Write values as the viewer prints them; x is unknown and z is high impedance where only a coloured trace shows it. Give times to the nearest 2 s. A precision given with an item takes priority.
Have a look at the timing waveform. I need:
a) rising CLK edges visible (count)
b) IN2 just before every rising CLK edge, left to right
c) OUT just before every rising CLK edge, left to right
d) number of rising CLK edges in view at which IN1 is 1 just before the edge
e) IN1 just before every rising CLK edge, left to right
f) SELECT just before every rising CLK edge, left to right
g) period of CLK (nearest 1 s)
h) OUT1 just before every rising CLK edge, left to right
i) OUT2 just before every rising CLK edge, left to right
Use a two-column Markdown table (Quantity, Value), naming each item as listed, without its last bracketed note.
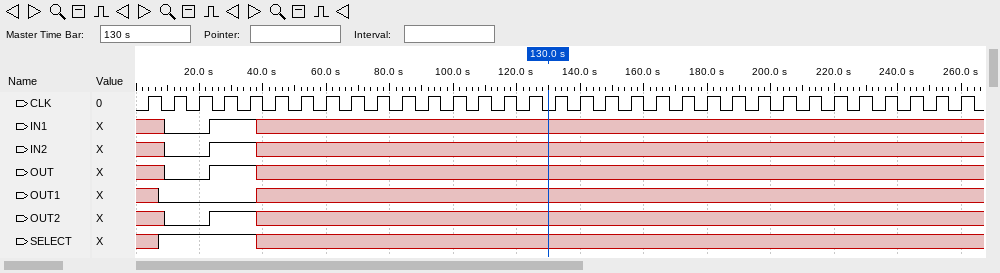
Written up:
| Quantity | Value |
|---|---|
| rising CLK edges visible | 33 |
| IN2 just before every rising CLK edge, left to right | x 0 0 1 1 x x x x x x x x x x x x x x x x x x x x x x x x x x x x |
| OUT just before every rising CLK edge, left to right | x 0 0 1 1 x x x x x x x x x x x x x x x x x x x x x x x x x x x x |
| number of rising CLK edges in view at which IN1 is 1 just before the edge | 2 |
| IN1 just before every rising CLK edge, left to right | x 0 0 1 1 x x x x x x x x x x x x x x x x x x x x x x x x x x x x |
| SELECT just before every rising CLK edge, left to right | x 1 1 1 1 x x x x x x x x x x x x x x x x x x x x x x x x x x x x |
| period of CLK | 8 s |
| OUT1 just before every rising CLK edge, left to right | x 0 0 0 0 x x x x x x x x x x x x x x x x x x x x x x x x x x x x |
| OUT2 just before every rising CLK edge, left to right | x 0 0 1 1 x x x x x x x x x x x x x x x x x x x x x x x x x x x x |
